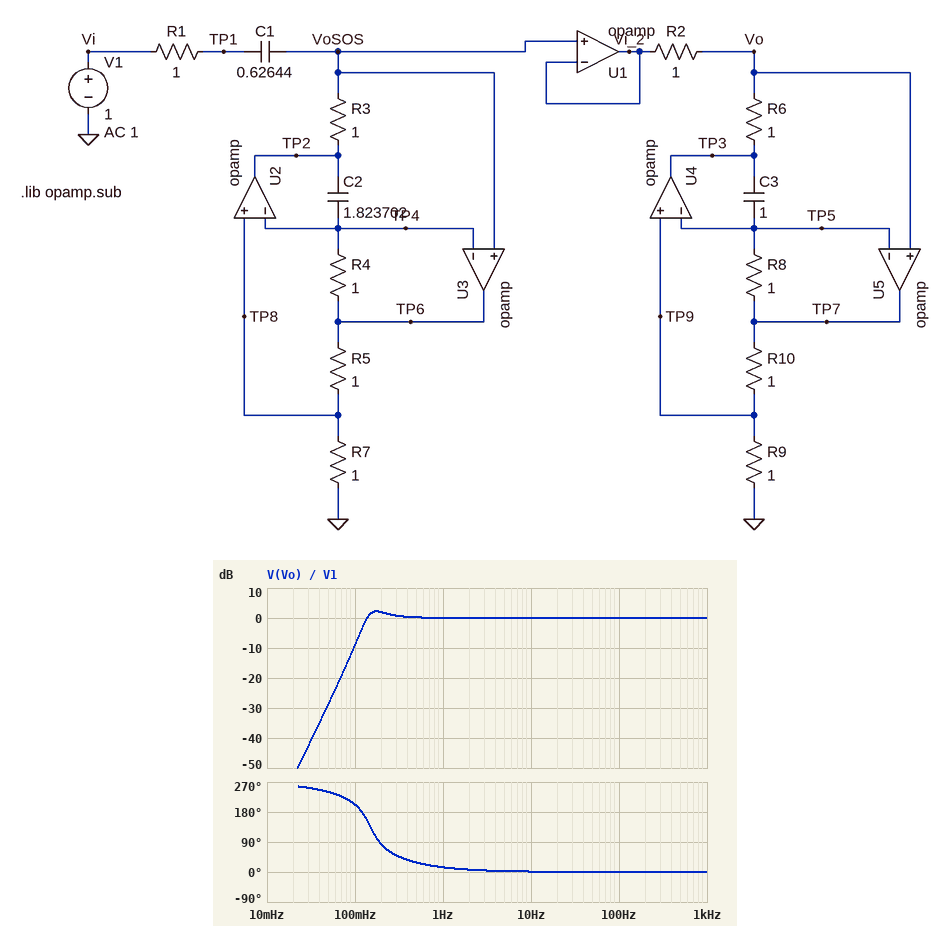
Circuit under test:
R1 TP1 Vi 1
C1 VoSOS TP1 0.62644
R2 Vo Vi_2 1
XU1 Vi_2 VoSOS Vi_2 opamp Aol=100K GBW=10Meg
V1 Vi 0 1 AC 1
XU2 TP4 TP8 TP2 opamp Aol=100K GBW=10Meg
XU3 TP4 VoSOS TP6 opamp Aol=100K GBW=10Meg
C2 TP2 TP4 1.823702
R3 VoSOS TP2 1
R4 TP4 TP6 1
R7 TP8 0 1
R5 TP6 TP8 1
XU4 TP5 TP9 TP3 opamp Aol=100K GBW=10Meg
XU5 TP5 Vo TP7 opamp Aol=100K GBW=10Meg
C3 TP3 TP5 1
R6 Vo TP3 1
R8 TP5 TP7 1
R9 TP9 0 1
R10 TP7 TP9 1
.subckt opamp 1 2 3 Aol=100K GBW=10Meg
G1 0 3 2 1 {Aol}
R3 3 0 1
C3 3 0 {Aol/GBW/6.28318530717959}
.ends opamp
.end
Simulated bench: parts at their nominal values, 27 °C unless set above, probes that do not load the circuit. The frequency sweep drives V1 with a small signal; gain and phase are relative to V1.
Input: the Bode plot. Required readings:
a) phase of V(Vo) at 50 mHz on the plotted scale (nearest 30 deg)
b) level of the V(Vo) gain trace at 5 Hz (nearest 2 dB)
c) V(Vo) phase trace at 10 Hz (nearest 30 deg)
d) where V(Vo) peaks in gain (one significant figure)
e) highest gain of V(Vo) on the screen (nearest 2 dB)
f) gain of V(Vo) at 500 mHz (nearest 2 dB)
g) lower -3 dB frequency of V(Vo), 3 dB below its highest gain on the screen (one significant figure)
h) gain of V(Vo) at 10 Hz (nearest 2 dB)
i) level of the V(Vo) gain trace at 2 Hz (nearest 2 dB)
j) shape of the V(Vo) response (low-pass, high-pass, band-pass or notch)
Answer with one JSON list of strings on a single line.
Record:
["240 deg", "0 dB", "0 deg", "200 mHz", "2 dB", "0 dB", "100 mHz", "0 dB", "0 dB", "high-pass"]
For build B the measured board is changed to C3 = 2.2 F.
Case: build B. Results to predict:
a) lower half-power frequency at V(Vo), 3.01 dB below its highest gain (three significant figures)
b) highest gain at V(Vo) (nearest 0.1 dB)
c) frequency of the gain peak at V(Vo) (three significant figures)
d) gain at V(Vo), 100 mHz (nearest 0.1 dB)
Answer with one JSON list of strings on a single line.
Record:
["129 mHz", "4.3 dB", "167 mHz", "-5.3 dB"]
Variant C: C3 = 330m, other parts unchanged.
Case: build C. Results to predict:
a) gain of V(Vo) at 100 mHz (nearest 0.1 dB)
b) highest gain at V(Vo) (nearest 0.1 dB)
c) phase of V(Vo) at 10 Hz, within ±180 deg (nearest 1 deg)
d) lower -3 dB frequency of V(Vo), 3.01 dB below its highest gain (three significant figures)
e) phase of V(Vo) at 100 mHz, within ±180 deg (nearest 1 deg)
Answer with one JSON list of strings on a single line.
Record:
["-17.4 dB", "0 dB", "3 deg", "382 mHz", "-137 deg"]
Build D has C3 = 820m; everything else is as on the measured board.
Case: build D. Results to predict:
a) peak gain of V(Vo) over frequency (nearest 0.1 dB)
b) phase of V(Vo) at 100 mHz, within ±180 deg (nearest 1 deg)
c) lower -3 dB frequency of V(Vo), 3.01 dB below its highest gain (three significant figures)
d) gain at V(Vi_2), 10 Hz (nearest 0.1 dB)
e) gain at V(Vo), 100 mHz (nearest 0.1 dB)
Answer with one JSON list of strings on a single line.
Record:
["1.4 dB", "-153 deg", "135 mHz", "0 dB", "-10.3 dB"]
